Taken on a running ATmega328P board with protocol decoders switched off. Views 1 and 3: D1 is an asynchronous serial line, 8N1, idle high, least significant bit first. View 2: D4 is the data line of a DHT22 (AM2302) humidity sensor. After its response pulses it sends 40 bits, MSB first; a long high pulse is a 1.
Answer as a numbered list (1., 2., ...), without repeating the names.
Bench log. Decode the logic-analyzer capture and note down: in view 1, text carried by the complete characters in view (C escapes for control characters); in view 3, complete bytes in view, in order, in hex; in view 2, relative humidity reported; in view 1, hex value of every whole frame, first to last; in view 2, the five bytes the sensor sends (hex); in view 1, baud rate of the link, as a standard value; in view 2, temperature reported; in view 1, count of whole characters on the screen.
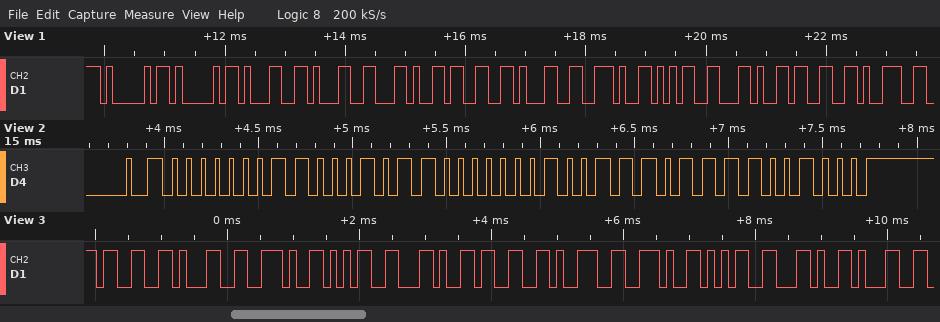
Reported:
1. "AA11,31.5,39"
2. 33 31 2E 35 2C 33 39 2E 35 2C 31
3. 39.5 %
4. 0x41 0x41 0x31 0x31 0x2C 0x33 0x31 0x2E 0x35 0x2C 0x33 0x39
5. 01 8B 01 3B C8
6. 9600 baud
7. 31.5 °C
8. 12
